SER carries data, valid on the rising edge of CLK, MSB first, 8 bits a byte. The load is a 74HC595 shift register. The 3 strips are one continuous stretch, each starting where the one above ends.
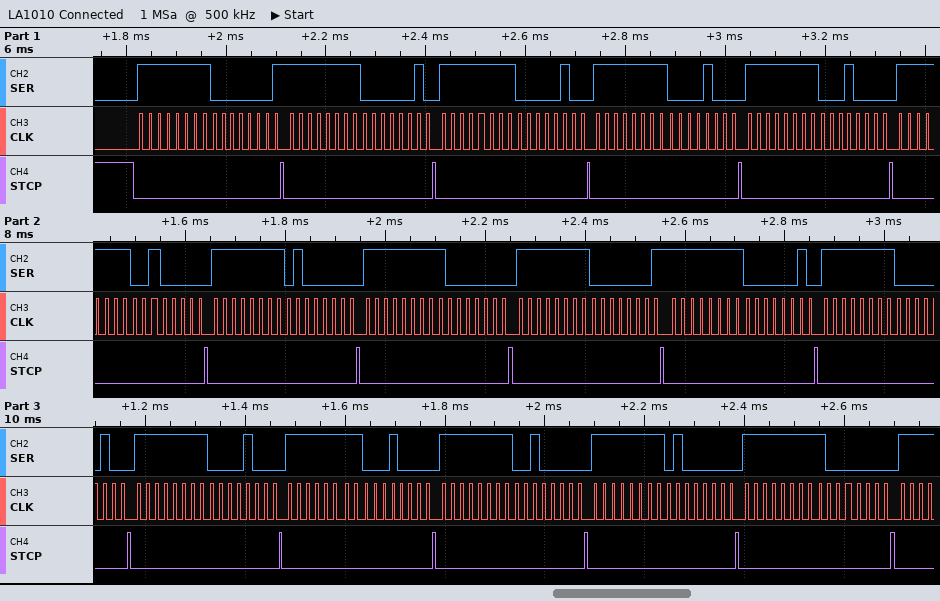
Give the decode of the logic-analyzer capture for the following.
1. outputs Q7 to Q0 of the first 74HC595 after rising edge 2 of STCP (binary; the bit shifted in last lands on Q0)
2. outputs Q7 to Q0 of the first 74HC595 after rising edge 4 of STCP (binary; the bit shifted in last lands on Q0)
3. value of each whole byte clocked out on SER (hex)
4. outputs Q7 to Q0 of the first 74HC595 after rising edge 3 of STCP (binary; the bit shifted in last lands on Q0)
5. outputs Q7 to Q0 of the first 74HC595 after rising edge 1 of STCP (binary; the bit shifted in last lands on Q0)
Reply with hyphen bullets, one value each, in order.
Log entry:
- 00000010
- 00001000
- 0xFF 0x01 0xFF 0x02 0xFF 0x04 0xFF 0x08 0xFF 0x10 0xFF 0x20 0xFF 0x40 0xFF 0x80 0xFF 0x01 0xFF 0x02 0xFF 0x04 0xFF 0x08 0xFF 0x10 0xFF 0x20 0xFF 0x40 0xFF 0x80
- 00000100
- 00000001
